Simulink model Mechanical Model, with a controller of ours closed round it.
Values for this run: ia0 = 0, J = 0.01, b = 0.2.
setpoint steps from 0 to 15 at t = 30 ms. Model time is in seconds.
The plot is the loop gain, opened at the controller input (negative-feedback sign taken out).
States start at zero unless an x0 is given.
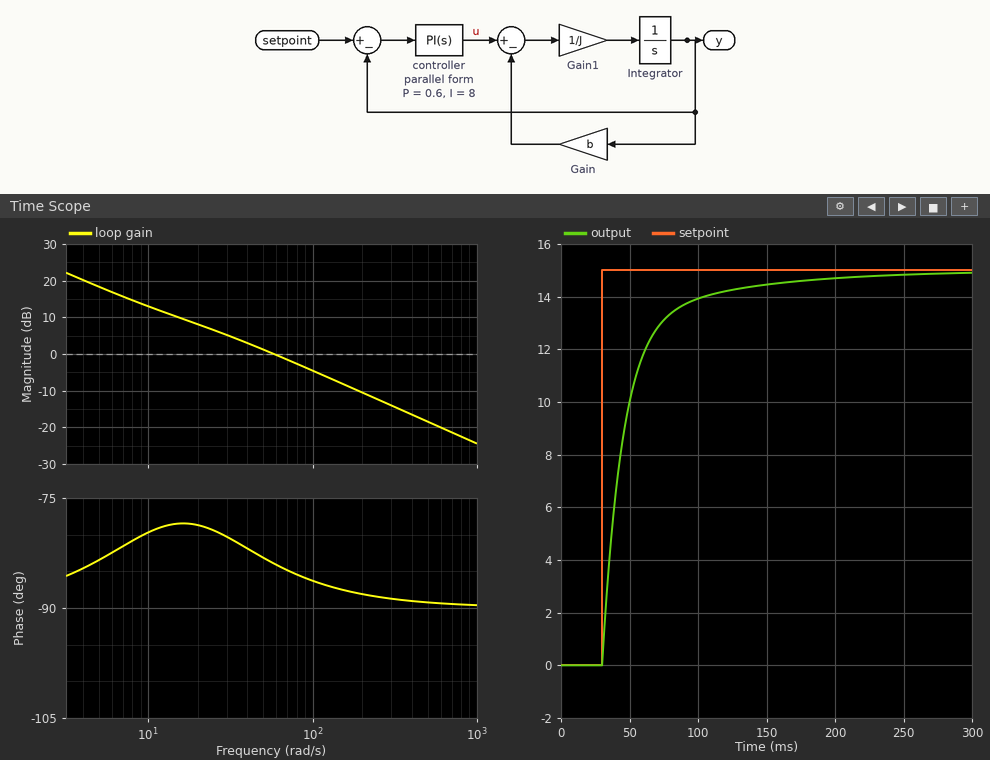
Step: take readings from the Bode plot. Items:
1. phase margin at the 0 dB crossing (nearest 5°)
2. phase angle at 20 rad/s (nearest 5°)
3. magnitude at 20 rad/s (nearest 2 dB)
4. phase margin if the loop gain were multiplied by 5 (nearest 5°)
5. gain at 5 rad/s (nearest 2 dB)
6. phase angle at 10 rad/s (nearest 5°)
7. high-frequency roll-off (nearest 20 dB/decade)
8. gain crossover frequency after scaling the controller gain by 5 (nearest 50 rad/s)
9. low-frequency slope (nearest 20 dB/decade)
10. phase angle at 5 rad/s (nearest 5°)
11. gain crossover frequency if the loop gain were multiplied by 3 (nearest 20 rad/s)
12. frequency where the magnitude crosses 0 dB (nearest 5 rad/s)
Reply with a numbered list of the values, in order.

1. 95°
2. -80°
3. 8 dB
4. 90°
5. 18 dB
6. -80°
7. -20 dB/decade
8. 300 rad/s
9. -20 dB/decade
10. -85°
11. 180 rad/s
12. 60 rad/s
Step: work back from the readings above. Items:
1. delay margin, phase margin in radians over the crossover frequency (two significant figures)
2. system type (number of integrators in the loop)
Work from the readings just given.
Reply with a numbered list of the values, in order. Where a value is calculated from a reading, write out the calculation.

1. 95 × π / 180 / 60 = 0.028 s
2. 1
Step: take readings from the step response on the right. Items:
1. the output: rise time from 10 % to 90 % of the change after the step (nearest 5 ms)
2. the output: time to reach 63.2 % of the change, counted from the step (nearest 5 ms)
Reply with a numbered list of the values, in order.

1. 50 ms
2. 20 ms
